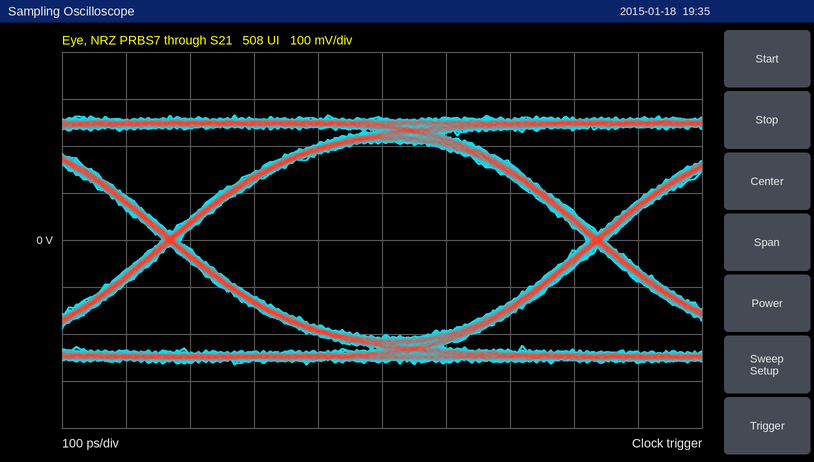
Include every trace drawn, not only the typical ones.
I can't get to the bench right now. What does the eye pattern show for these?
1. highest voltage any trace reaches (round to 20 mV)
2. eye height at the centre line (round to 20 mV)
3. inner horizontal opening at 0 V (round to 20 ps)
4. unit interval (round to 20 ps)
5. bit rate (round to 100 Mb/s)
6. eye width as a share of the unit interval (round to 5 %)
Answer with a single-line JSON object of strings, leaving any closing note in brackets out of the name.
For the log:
{"highest voltage any trace reaches": "260 mV", "eye height at the centre line": "420 mV", "inner horizontal opening at 0 V": "640 ps", "unit interval": "660 ps", "bit rate": "1.5 Gb/s", "eye width as a share of the unit interval": "95 %"}
